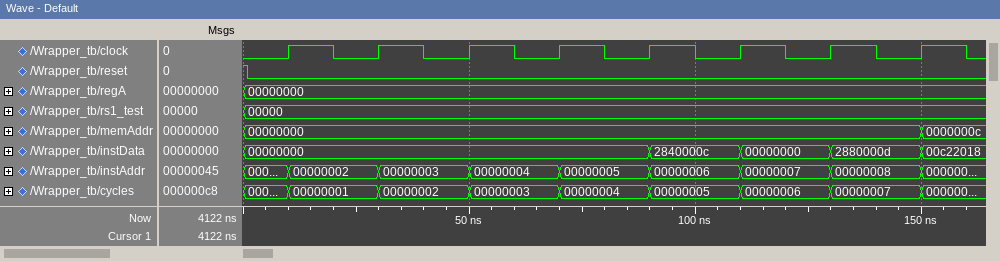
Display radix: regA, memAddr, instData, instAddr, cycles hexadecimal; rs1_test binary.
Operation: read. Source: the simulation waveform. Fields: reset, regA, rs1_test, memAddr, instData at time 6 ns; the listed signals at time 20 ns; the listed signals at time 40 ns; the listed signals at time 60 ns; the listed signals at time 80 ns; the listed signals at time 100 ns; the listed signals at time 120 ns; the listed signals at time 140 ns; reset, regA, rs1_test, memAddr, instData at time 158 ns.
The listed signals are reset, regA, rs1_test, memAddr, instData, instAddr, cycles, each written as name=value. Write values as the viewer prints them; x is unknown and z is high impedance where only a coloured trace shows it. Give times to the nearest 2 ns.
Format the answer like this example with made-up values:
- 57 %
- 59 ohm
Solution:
- reset=0, regA=00000000, rs1_test=00000, memAddr=00000000, instData=00000000
- reset=0, regA=00000000, rs1_test=00000, memAddr=00000000, instData=00000000, instAddr=00000002, cycles=00000001
- reset=0, regA=00000000, rs1_test=00000, memAddr=00000000, instData=00000000, instAddr=00000003, cycles=00000002
- reset=0, regA=00000000, rs1_test=00000, memAddr=00000000, instData=00000000, instAddr=00000004, cycles=00000003
- reset=0, regA=00000000, rs1_test=00000, memAddr=00000000, instData=00000000, instAddr=00000005, cycles=00000004
- reset=0, regA=00000000, rs1_test=00000, memAddr=00000000, instData=2840000c, instAddr=00000006, cycles=00000005
- reset=0, regA=00000000, rs1_test=00000, memAddr=00000000, instData=00000000, instAddr=00000007, cycles=00000006
- reset=0, regA=00000000, rs1_test=00000, memAddr=00000000, instData=2880000d, instAddr=00000008, cycles=00000007
- reset=0, regA=00000000, rs1_test=00000, memAddr=0000000c, instData=00c22018
